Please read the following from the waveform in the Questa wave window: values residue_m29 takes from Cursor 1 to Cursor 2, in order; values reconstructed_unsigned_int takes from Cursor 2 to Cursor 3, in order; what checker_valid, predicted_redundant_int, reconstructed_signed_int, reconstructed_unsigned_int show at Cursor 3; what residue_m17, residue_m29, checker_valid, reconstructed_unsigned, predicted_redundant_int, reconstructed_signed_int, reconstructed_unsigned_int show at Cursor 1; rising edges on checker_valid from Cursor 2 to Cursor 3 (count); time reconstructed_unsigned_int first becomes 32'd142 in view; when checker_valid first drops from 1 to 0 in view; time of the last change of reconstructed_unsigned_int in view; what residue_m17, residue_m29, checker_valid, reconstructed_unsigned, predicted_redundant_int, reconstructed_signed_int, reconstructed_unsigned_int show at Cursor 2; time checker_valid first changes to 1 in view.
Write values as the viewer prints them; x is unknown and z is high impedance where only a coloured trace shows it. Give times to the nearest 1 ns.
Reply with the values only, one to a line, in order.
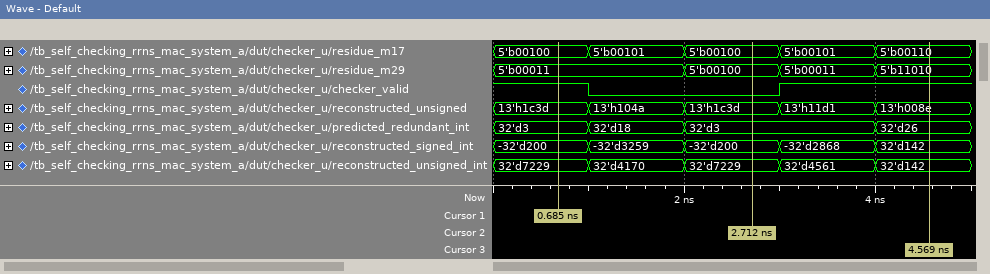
5'b00011, 5'b00100
32'd7229, 32'd4561, 32'd142
checker_valid=1, predicted_redundant_int=32'd26, reconstructed_signed_int=32'd142, reconstructed_unsigned_int=32'd142
residue_m17=5'b00100, residue_m29=5'b00011, checker_valid=1, reconstructed_unsigned=13'h1c3d, predicted_redundant_int=32'd3, reconstructed_signed_int=-32'd200, reconstructed_unsigned_int=32'd7229
1
4 ns
1 ns
4 ns
residue_m17=5'b00100, residue_m29=5'b00100, checker_valid=0, reconstructed_unsigned=13'h1c3d, predicted_redundant_int=32'd3, reconstructed_signed_int=-32'd200, reconstructed_unsigned_int=32'd7229
3 ns
